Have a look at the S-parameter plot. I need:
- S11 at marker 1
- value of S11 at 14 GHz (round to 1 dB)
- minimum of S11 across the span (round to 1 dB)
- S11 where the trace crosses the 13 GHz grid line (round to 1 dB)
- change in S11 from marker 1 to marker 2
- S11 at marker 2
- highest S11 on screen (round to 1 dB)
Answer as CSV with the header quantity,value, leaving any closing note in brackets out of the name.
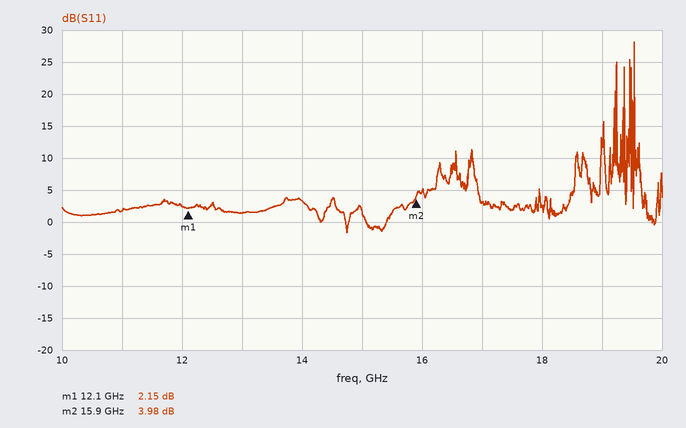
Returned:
quantity,value
S11 at marker 1,2.15 dB
value of S11 at 14 GHz,3 dB
minimum of S11 across the span,-2 dB
S11 where the trace crosses the 13 GHz grid line,1 dB
change in S11 from marker 1 to marker 2,1.83 dB
S11 at marker 2,3.98 dB
highest S11 on screen,28 dB
